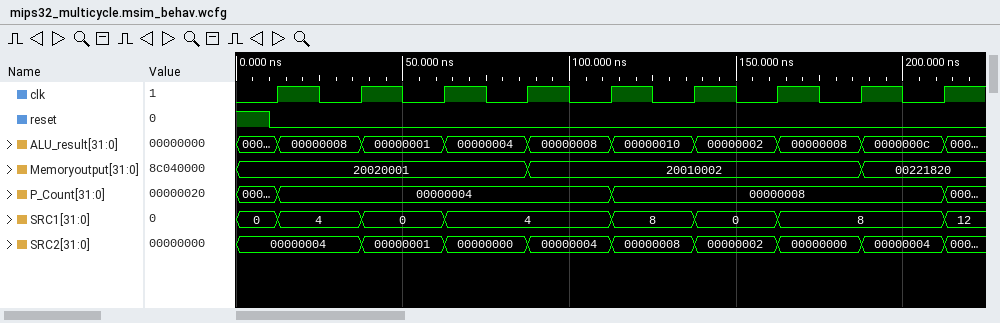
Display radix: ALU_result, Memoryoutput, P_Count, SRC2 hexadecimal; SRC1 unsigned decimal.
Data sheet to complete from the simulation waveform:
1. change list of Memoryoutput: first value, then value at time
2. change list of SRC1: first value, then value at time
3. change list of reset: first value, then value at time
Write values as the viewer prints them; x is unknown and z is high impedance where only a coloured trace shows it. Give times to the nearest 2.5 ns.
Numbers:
20020001, 20010002 at 87.5 ns, 00221820 at 187.5 ns
0, 4 at 12.5 ns, 0 at 37.5 ns, 4 at 62.5 ns, 8 at 112.5 ns, 0 at 137.5 ns, 8 at 162.5 ns, 12 at 212.5 ns
1, 0 at 10 ns
